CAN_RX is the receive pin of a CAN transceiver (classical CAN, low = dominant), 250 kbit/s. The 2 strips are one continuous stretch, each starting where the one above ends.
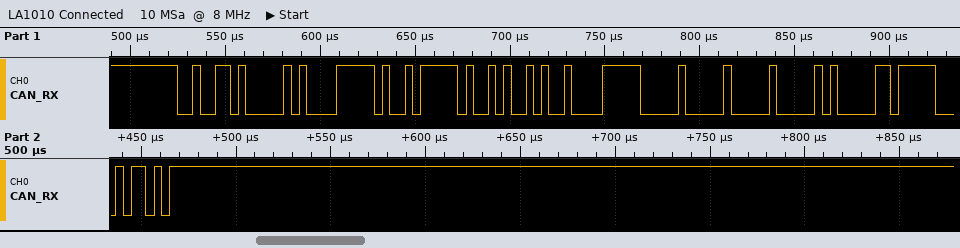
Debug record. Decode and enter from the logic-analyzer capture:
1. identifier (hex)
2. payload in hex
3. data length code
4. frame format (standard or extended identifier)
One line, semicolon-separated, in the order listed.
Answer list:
0x268; 7E 5F 94 A4 3E 00 00 10; 8; standard
